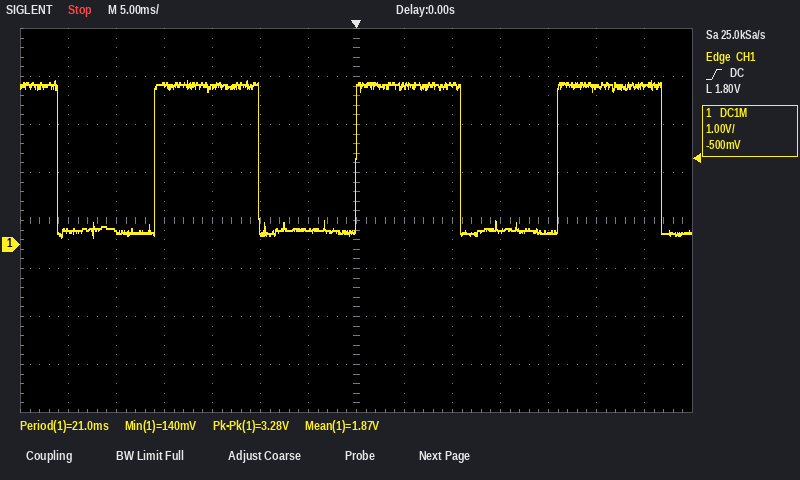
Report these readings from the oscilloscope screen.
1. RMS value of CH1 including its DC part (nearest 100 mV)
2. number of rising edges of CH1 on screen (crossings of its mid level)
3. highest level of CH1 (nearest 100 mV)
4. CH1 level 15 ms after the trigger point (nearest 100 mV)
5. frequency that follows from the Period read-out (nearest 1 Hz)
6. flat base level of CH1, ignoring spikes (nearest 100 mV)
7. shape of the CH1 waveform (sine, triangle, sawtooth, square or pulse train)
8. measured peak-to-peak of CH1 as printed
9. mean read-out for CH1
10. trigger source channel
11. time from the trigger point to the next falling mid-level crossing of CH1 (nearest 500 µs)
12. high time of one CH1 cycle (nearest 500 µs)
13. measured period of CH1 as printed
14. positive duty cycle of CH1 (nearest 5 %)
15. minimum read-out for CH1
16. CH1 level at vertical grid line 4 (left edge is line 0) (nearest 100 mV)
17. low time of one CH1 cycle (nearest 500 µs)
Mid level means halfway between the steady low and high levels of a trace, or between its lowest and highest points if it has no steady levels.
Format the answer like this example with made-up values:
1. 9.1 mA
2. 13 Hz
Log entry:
1. 2.4 V
2. 3
3. 3.4 V
4. 300 mV
5. 48 Hz
6. 300 mV
7. square
8. 3.28 V
9. 1.87 V
10. CH1
11. 11.0 ms
12. 11.0 ms
13. 21.0 ms
14. 50 %
15. 140 mV
16. 3.3 V
17. 10.0 ms
